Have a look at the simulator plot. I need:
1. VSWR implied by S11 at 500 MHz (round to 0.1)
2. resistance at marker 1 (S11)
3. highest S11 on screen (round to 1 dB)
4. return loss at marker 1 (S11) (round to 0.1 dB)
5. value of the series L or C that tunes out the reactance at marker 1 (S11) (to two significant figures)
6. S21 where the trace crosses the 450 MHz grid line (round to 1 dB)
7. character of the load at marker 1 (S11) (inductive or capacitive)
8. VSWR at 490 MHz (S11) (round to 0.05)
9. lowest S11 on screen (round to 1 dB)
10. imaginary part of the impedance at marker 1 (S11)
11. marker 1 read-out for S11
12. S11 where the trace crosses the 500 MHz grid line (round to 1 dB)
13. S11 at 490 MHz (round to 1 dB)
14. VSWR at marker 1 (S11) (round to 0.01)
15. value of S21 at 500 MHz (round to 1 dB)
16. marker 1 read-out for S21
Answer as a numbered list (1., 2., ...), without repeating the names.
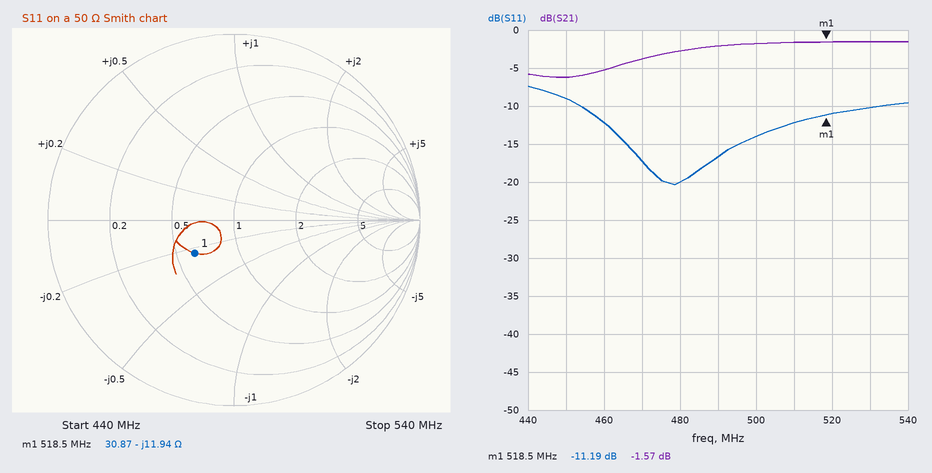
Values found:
1. 1.5
2. 30.87 Ω
3. -7 dB
4. 11.2 dB
5. 3.7 nH
6. -6 dB
7. capacitive
8. 1.35
9. -20 dB
10. -11.94 Ω
11. -11.19 dB
12. -14 dB
13. -17 dB
14. 1.76
15. -2 dB
16. -1.57 dB
